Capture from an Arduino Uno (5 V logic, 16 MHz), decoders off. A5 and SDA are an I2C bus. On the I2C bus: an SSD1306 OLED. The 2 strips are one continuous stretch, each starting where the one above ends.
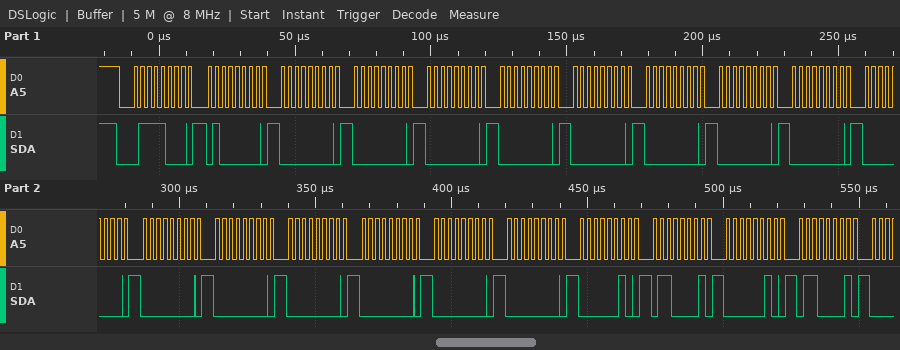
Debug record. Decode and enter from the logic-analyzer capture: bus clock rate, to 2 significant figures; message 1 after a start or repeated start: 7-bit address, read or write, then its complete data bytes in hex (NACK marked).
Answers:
400 kHz
0x3C write: 40 00 00 00 00 00 00 00 00 00 00 00 00 00 00 00 02 61 02 61
